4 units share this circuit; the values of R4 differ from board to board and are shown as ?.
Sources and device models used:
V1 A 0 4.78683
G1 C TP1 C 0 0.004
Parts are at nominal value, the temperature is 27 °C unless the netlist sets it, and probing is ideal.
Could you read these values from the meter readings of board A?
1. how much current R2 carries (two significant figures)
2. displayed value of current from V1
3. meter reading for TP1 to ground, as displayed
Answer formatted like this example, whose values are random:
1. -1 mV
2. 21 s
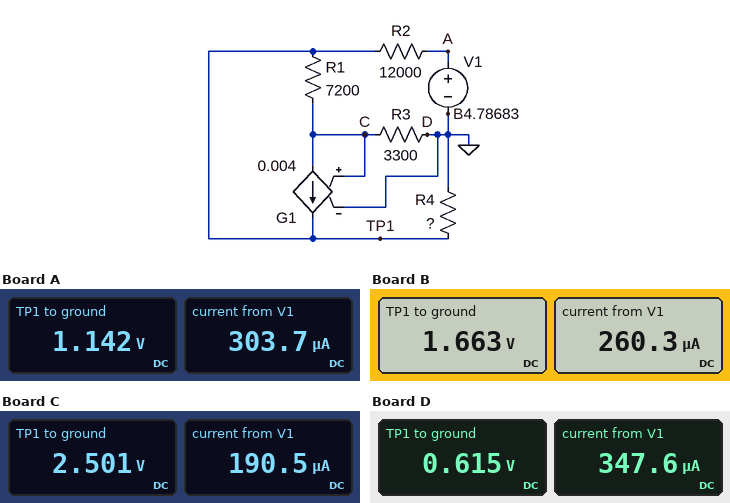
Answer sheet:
1. 300 µA
2. 303.7 µA
3. 1.142 V
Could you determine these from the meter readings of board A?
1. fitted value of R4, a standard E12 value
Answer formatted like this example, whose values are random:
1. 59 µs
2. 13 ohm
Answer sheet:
1. 3.9 kΩ
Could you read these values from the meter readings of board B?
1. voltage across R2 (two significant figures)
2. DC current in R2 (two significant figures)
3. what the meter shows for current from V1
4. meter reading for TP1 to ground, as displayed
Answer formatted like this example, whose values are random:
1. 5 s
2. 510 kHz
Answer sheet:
1. 3.1 V
2. 260 µA
3. 260.3 µA
4. 1.663 V
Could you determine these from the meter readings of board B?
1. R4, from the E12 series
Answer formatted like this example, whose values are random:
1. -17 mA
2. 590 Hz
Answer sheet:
1. 6.8 kΩ
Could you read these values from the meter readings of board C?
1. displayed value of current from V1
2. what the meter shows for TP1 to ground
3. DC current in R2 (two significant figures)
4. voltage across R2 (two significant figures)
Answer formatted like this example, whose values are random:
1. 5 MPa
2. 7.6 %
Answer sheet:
1. 190.5 µA
2. 2.501 V
3. 190 µA
4. 2.3 V
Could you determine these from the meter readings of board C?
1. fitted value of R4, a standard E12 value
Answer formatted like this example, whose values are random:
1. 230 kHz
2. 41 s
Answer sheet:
1. 15 kΩ
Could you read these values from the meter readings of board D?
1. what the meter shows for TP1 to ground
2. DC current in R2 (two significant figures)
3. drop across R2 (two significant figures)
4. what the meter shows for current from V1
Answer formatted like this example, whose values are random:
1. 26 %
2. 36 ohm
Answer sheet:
1. 0.615 V
2. 350 µA
3. 4.2 V
4. 347.6 µA
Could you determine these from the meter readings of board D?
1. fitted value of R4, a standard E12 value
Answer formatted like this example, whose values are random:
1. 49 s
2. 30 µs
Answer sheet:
1. 1.8 kΩ
